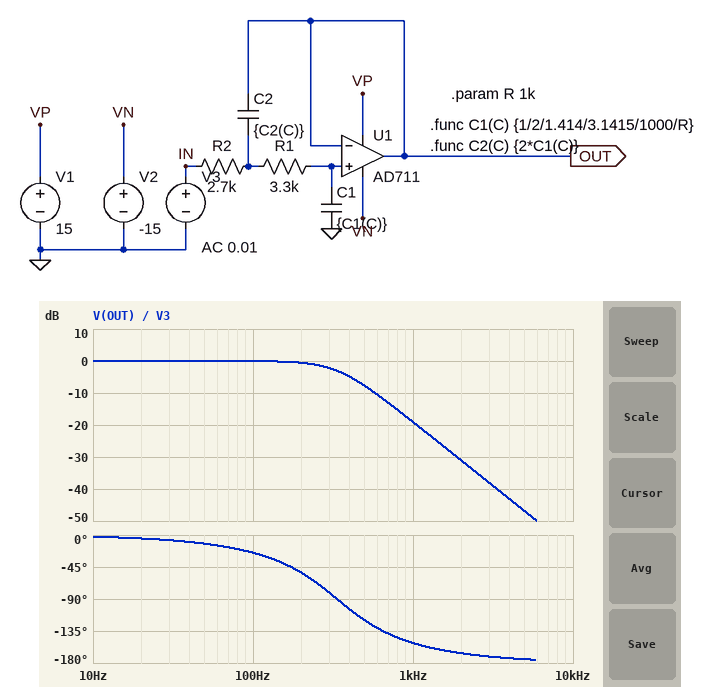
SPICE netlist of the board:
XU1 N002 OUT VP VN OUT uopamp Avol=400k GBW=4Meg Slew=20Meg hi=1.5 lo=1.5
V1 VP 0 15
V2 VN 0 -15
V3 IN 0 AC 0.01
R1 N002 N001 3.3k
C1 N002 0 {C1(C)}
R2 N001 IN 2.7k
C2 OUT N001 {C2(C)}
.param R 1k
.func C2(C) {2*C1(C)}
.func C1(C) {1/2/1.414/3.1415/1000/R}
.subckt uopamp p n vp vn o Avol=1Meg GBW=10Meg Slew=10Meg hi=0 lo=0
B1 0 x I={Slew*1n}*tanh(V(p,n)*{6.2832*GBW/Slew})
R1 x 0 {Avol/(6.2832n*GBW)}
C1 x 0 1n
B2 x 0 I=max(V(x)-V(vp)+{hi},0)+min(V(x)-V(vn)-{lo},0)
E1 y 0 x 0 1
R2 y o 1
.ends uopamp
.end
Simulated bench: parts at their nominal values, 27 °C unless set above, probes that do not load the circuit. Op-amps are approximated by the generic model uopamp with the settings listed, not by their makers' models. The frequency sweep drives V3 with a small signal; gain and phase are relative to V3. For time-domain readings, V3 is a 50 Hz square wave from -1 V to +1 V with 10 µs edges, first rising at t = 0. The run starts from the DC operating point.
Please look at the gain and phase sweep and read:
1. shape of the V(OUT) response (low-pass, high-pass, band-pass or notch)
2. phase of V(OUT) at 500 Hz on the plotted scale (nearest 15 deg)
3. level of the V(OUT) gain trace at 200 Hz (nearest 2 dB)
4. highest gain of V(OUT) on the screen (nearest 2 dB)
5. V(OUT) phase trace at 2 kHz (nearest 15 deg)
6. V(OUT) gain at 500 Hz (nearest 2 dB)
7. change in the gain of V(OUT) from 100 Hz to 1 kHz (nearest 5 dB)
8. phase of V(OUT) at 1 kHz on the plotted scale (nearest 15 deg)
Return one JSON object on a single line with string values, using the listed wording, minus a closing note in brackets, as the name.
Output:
{"shape of the V(OUT) response": "low-pass", "phase of V(OUT) at 500 Hz on the plotted scale": "-120 deg", "level of the V(OUT) gain trace at 200 Hz": "0 dB", "highest gain of V(OUT) on the screen": "0 dB", "V(OUT) phase trace at 2 kHz": "-165 deg", "V(OUT) gain at 500 Hz": "-8 dB", "change in the gain of V(OUT) from 100 Hz to 1 kHz": "-20 dB", "phase of V(OUT) at 1 kHz on the plotted scale": "-150 deg"}
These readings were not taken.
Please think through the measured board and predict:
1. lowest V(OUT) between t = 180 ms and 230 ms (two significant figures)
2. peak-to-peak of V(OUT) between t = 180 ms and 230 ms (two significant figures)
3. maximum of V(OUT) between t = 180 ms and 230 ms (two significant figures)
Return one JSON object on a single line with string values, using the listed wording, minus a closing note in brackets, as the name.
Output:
{"lowest V(OUT) between t = 180 ms and 230 ms": "-1.1 V", "peak-to-peak of V(OUT) between t = 180 ms and 230 ms": "2.2 V", "maximum of V(OUT) between t = 180 ms and 230 ms": "1.1 V"}
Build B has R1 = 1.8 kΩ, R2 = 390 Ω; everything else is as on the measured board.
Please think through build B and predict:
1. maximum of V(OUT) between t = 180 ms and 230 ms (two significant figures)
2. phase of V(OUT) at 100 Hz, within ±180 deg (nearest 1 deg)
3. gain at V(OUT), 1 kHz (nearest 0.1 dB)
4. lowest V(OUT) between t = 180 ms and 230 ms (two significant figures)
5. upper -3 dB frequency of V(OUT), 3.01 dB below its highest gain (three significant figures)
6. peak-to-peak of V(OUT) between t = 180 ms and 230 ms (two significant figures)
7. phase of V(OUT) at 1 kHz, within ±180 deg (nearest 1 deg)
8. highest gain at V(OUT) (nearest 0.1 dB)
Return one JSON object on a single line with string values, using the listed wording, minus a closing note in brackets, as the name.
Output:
{"maximum of V(OUT) between t = 180 ms and 230 ms": "1.0 V", "phase of V(OUT) at 100 Hz, within ±180 deg": "-9 deg", "gain at V(OUT), 1 kHz": "-4.0 dB", "lowest V(OUT) between t = 180 ms and 230 ms": "-1.0 V", "upper -3 dB frequency of V(OUT), 3.01 dB below its highest gain": "858 Hz", "peak-to-peak of V(OUT) between t = 180 ms and 230 ms": "2.0 V", "phase of V(OUT) at 1 kHz, within ±180 deg": "-79 deg", "highest gain at V(OUT)": "0 dB"}
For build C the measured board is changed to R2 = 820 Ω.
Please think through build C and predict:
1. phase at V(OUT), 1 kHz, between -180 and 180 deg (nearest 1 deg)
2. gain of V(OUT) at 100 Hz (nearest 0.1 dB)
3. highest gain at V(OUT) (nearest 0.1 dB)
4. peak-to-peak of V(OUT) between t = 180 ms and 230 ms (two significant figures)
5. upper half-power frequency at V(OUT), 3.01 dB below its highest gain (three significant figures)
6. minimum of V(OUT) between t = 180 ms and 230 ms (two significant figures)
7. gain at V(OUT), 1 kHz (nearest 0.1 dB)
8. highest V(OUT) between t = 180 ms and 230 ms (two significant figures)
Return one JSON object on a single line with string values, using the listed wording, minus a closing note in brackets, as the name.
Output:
{"phase at V(OUT), 1 kHz, between -180 and 180 deg": "-120 deg", "gain of V(OUT) at 100 Hz": "-0.1 dB", "highest gain at V(OUT)": "0 dB", "peak-to-peak of V(OUT) between t = 180 ms and 230 ms": "2.0 V", "upper half-power frequency at V(OUT), 3.01 dB below its highest gain": "464 Hz", "minimum of V(OUT) between t = 180 ms and 230 ms": "-1.0 V", "gain at V(OUT), 1 kHz": "-10.6 dB", "highest V(OUT) between t = 180 ms and 230 ms": "1.0 V"}
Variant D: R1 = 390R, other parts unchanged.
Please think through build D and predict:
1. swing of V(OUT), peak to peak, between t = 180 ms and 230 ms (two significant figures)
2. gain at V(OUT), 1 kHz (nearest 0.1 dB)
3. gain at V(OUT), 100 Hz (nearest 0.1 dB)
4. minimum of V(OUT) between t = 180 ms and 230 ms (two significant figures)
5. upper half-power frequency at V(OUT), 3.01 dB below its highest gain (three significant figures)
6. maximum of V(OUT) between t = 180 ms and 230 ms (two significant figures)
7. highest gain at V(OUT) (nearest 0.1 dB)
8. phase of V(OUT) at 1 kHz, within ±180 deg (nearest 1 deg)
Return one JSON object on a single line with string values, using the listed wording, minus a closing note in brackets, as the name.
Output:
{"swing of V(OUT), peak to peak, between t = 180 ms and 230 ms": "2.0 V", "gain at V(OUT), 1 kHz": "-6.8 dB", "gain at V(OUT), 100 Hz": "-0.1 dB", "minimum of V(OUT) between t = 180 ms and 230 ms": "-1.0 V", "upper half-power frequency at V(OUT), 3.01 dB below its highest gain": "574 Hz", "maximum of V(OUT) between t = 180 ms and 230 ms": "1.0 V", "highest gain at V(OUT)": "0 dB", "phase of V(OUT) at 1 kHz, within ±180 deg": "-91 deg"}
